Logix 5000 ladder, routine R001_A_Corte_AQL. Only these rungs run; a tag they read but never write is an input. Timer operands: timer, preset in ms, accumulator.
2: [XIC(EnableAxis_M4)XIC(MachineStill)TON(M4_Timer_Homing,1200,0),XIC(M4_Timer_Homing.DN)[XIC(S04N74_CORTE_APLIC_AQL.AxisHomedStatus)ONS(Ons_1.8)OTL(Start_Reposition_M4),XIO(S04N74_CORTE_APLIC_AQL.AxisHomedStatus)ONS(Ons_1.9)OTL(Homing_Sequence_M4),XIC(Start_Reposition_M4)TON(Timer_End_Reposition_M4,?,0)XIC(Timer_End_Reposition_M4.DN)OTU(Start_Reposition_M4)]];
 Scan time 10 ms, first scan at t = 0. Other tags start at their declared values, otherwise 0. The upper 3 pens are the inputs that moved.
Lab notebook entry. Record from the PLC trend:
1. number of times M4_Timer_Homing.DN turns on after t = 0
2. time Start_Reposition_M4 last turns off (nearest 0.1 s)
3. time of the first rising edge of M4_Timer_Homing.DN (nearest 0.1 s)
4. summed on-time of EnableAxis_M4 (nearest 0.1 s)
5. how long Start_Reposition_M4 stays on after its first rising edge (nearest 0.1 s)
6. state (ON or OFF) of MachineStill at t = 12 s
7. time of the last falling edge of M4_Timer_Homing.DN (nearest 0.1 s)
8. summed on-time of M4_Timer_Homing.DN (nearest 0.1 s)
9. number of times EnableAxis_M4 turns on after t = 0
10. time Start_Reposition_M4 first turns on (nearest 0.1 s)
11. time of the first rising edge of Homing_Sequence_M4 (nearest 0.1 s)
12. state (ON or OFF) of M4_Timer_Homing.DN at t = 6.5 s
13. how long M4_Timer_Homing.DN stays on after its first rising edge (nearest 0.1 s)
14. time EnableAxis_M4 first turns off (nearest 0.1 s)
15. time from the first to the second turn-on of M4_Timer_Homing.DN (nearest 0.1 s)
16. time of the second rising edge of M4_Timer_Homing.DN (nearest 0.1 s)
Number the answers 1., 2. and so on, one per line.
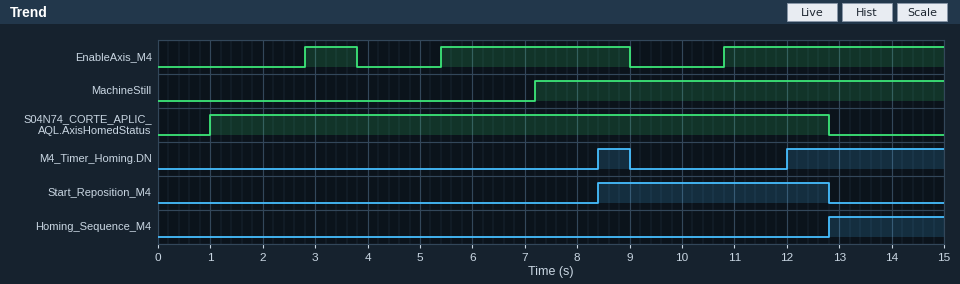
1. 2
2. 12.8 s
3. 8.4 s
4. 8.8 s
5. 4.4 s
6. ON
7. 9.0 s
8. 3.6 s
9. 3
10. 8.4 s
11. 12.8 s
12. OFF
13. 0.6 s
14. 3.8 s
15. 3.6 s
16. 12.0 s
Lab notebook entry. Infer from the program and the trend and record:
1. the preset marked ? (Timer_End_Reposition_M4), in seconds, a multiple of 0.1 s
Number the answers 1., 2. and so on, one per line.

1. 0.8 s
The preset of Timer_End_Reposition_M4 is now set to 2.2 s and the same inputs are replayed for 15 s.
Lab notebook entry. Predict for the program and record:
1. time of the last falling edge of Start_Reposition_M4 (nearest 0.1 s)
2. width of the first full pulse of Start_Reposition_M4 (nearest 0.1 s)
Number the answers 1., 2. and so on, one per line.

1. 14.2 s
2. 5.8 s
